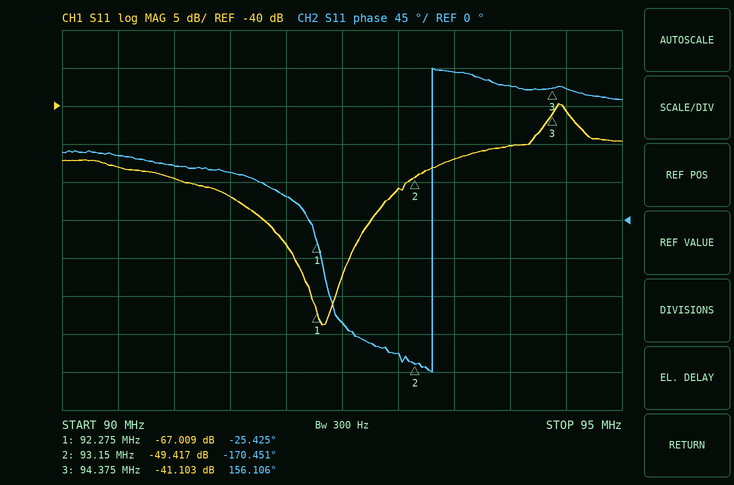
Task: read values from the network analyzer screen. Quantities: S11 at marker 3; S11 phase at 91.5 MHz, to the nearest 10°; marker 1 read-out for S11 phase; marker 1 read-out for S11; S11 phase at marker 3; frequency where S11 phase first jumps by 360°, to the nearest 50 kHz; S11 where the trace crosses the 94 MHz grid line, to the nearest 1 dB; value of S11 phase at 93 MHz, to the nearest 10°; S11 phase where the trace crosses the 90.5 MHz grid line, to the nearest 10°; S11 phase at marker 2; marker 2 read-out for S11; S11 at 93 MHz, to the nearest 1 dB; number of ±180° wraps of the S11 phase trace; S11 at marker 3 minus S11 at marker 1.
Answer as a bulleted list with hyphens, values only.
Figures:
- -41.103 dB
- 60°
- -25.425°
- -67.009 dB
- 156.106°
- 93.30 MHz
- -45 dB
- -160°
- 80°
- -170.451°
- -49.417 dB
- -51 dB
- 1
- 25.906 dB
